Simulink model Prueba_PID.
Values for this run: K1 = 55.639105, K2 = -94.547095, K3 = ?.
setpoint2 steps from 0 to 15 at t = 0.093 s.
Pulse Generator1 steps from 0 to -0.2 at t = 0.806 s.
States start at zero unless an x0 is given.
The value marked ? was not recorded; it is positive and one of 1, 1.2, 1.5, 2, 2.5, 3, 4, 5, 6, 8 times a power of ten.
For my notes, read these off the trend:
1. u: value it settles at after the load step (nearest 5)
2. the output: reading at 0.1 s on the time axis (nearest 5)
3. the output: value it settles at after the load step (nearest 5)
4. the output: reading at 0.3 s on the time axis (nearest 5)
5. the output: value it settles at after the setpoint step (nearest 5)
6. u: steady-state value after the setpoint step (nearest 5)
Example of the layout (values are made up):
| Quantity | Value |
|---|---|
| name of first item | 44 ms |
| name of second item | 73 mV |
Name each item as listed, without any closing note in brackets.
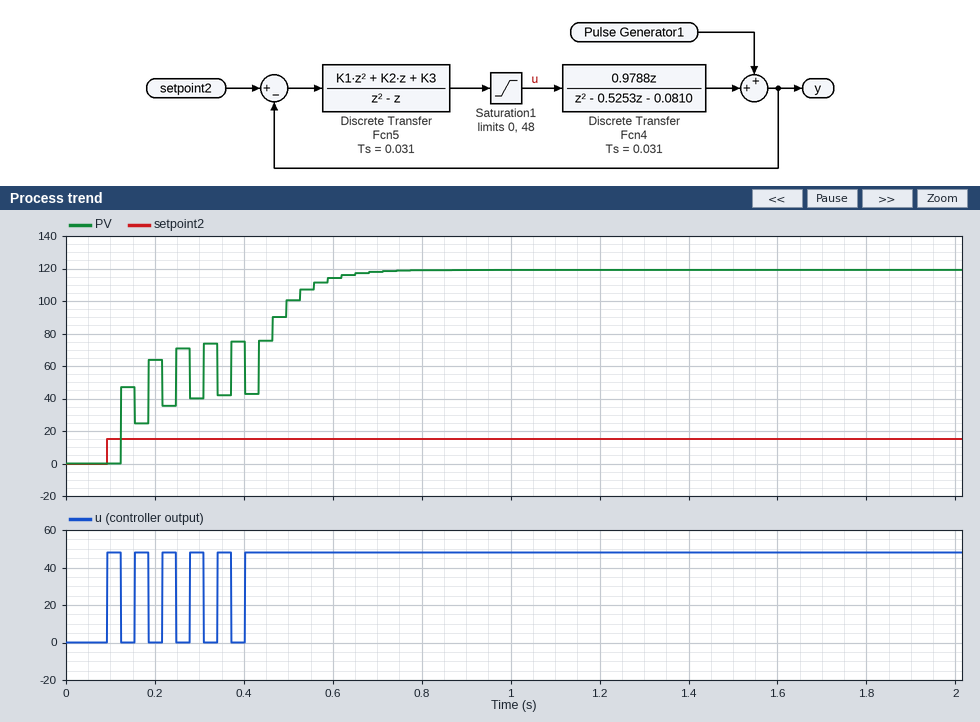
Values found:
| Quantity | Value |
|---|---|
| u: value it settles at after the load step | 50 |
| the output: reading at 0.1 s on the time axis | 0 |
| the output: value it settles at after the load step | 120 |
| the output: reading at 0.3 s on the time axis | 40 |
| the output: value it settles at after the setpoint step | 120 |
| u: steady-state value after the setpoint step | 50 |
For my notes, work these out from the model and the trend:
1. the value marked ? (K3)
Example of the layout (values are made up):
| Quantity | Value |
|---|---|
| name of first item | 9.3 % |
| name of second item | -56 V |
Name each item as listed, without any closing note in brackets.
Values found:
| Quantity | Value |
|---|---|
| the value marked ? | 30 |
